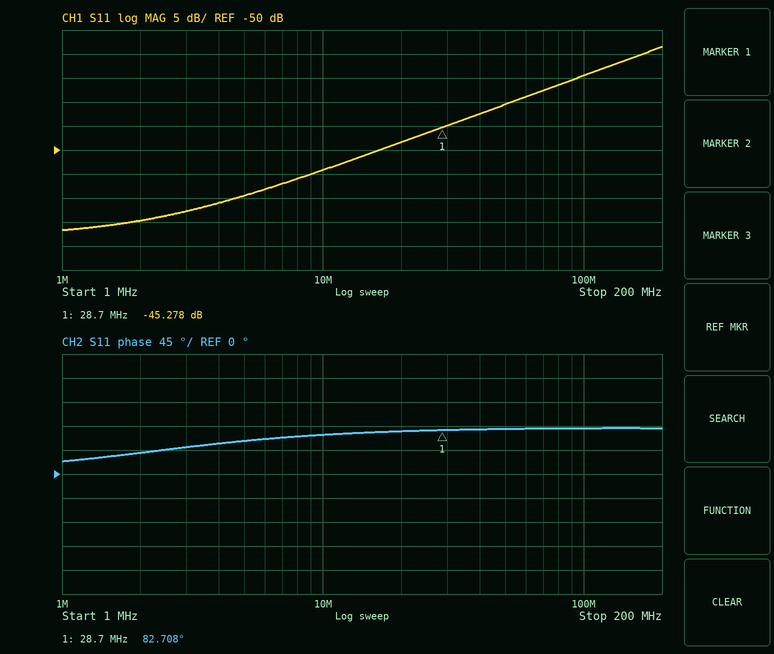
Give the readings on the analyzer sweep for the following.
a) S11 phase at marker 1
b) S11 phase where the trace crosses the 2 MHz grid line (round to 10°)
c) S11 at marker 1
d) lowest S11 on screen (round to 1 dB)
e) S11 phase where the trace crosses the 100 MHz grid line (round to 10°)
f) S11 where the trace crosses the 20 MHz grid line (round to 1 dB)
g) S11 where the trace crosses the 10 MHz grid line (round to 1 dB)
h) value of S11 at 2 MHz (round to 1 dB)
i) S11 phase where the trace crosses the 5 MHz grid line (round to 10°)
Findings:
82.708°
40°
-45.278 dB
-67 dB
90°
-48 dB
-54 dB
-65 dB
60°
